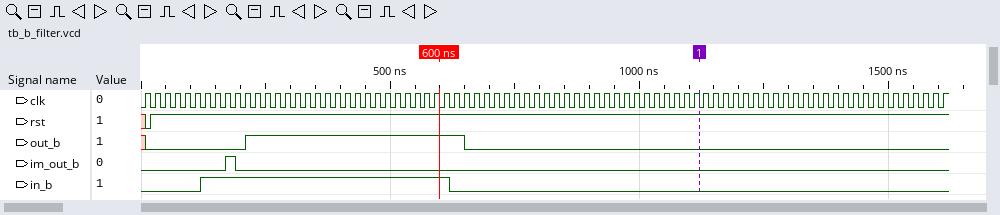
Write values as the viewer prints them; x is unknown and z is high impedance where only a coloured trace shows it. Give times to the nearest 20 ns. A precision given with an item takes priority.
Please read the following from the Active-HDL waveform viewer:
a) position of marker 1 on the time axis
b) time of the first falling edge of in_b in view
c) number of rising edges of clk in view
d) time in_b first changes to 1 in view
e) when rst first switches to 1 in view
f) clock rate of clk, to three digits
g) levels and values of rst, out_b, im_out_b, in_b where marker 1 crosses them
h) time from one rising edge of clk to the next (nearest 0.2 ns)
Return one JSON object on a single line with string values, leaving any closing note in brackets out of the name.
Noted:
{"position of marker 1 on the time axis": "1120 ns", "time of the first falling edge of in_b in view": "620 ns", "number of rising edges of clk in view": "81", "time in_b first changes to 1 in view": "120 ns", "when rst first switches to 1 in view": "20 ns", "clock rate of clk, to three digits": "50.0 MHz", "levels and values of rst, out_b, im_out_b, in_b where marker 1 crosses them": "rst=1, out_b=0, im_out_b=0, in_b=0", "time from one rising edge of clk to the next": "20 ns"}
